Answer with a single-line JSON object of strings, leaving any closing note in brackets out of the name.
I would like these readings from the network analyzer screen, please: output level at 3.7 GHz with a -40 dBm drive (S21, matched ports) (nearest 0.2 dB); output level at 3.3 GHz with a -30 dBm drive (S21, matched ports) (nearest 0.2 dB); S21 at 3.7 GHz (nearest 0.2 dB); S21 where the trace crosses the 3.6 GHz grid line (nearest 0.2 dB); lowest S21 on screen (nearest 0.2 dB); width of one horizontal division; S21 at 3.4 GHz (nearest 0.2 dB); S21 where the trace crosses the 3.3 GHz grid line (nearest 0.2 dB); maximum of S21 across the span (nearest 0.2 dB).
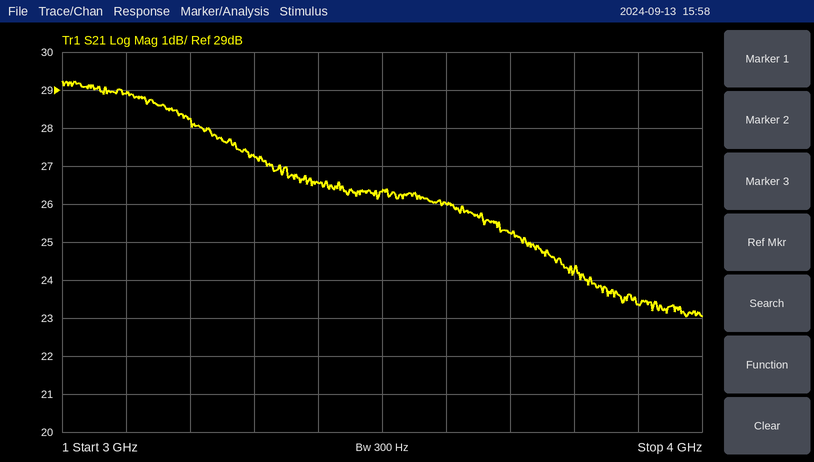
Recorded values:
{"output level at 3.7 GHz with a -40 dBm drive (S21, matched ports)": "-14.8 dBm", "output level at 3.3 GHz with a -30 dBm drive (S21, matched ports)": "-2.8 dBm", "S21 at 3.7 GHz": "25.2 dB", "S21 where the trace crosses the 3.6 GHz grid line": "26.0 dB", "lowest S21 on screen": "23.0 dB", "width of one horizontal division": "100 MHz", "S21 at 3.4 GHz": "26.6 dB", "S21 where the trace crosses the 3.3 GHz grid line": "27.2 dB", "maximum of S21 across the span": "29.2 dB"}
